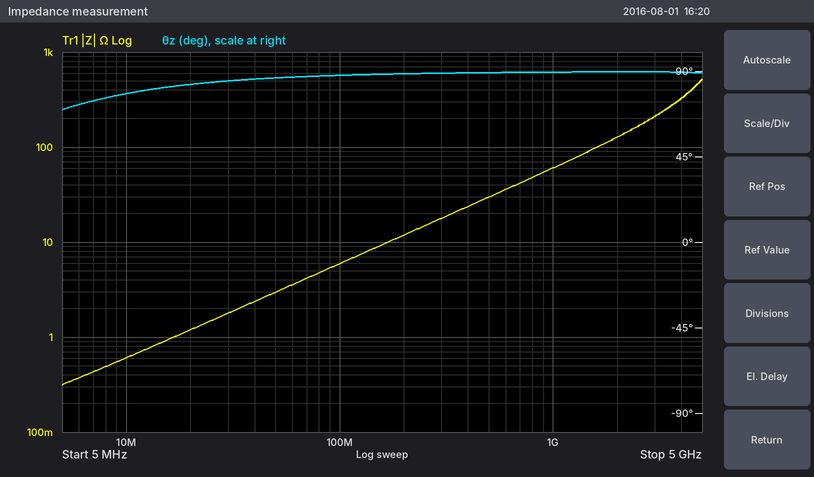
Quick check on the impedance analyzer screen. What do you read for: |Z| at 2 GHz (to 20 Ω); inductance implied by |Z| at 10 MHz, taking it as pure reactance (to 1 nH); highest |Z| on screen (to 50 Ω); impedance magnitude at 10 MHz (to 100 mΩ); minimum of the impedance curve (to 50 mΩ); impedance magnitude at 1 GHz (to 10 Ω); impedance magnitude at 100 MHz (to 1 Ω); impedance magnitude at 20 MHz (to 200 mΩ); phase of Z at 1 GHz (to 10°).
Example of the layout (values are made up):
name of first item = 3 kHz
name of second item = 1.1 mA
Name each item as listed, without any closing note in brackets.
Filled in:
|Z| at 2 GHz = 120 Ω
inductance implied by |Z| at 10 MHz, taking it as pure reactance = 10 nH
highest |Z| on screen = 500 Ω
impedance magnitude at 10 MHz = 600 mΩ
minimum of the impedance curve = 300 mΩ
impedance magnitude at 1 GHz = 60 Ω
impedance magnitude at 100 MHz = 6 Ω
impedance magnitude at 20 MHz = 1.2 Ω
phase of Z at 1 GHz = 90°
